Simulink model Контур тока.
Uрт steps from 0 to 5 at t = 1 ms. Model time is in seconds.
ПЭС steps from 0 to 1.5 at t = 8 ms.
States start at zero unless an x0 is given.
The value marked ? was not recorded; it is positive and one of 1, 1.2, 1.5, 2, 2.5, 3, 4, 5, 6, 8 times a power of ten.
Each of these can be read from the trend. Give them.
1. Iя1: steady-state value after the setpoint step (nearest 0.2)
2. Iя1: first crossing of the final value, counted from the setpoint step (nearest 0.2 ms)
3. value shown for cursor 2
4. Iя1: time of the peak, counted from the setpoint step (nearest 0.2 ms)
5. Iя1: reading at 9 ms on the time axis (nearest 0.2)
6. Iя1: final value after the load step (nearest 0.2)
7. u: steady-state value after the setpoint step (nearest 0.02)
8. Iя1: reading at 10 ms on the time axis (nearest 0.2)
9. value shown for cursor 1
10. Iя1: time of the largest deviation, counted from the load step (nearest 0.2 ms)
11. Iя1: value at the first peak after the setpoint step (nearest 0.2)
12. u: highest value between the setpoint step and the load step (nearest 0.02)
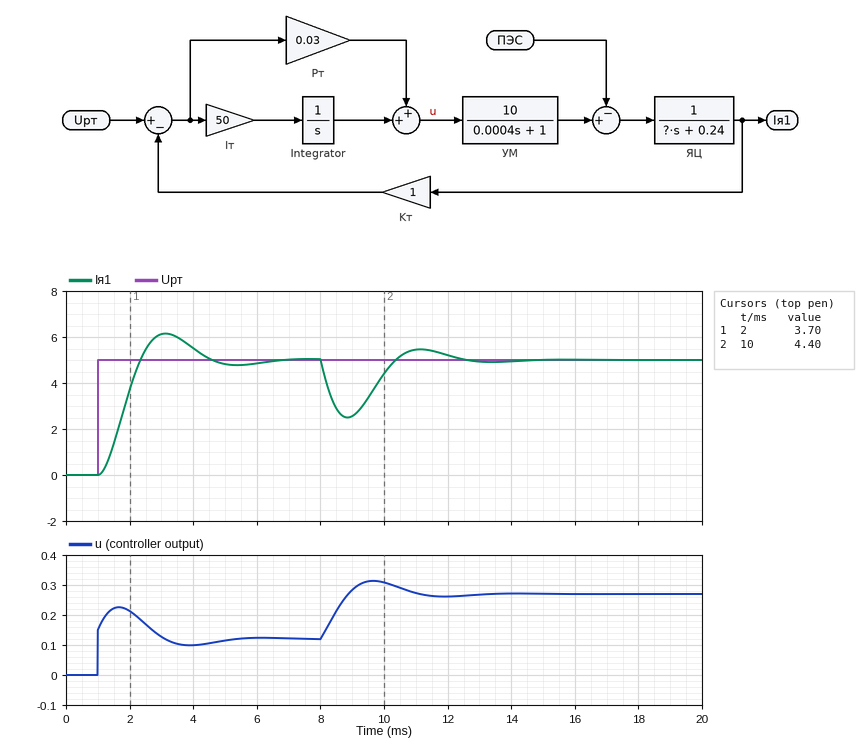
5.0
1.4 ms
4.40
2.2 ms
2.6
5.0
0.12
4.4
3.70
0.8 ms
6.2
0.22
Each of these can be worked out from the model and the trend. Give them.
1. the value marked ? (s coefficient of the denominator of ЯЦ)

0.00025
